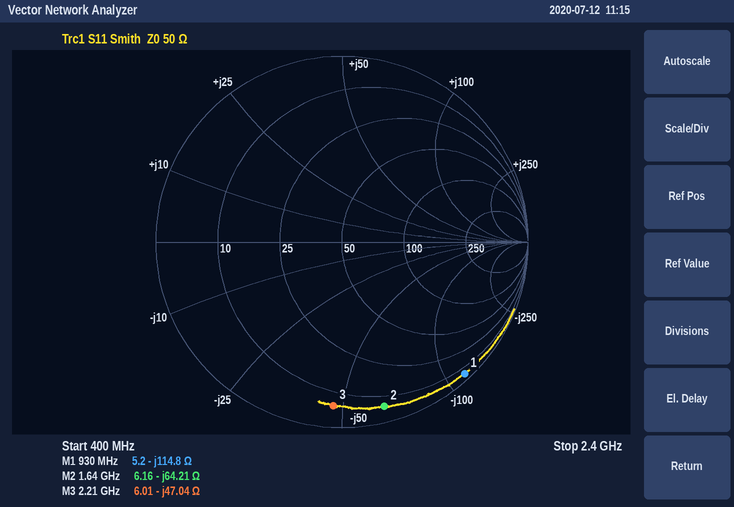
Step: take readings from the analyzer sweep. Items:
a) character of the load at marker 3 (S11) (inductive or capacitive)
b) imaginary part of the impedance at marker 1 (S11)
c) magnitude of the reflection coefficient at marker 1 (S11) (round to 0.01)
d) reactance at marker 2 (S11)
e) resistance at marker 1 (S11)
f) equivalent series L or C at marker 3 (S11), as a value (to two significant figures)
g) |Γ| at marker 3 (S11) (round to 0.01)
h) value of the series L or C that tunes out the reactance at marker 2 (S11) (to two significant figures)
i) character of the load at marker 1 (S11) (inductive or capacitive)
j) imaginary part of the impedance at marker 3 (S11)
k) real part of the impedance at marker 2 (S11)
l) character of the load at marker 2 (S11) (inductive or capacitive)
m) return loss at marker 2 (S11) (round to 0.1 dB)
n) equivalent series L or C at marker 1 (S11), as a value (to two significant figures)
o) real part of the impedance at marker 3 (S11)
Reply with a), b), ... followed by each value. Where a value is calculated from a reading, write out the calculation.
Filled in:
a) capacitive
b) -114.8 Ω
c) 0.97
d) -64.21 Ω
e) 5.2 Ω
f) C = 1/(2π × 2.21 GHz × 47.04 Ω) ≈ 1.5 pF
g) 0.88
h) L = 64.21 Ω/(2π × 1.64 GHz) ≈ 6.2 nH
i) capacitive
j) -47.04 Ω
k) 6.16 Ω
l) capacitive
m) 0.8 dB
n) C = 1/(2π × 930 MHz × 114.8 Ω) ≈ 1.5 pF
o) 6.01 Ω
